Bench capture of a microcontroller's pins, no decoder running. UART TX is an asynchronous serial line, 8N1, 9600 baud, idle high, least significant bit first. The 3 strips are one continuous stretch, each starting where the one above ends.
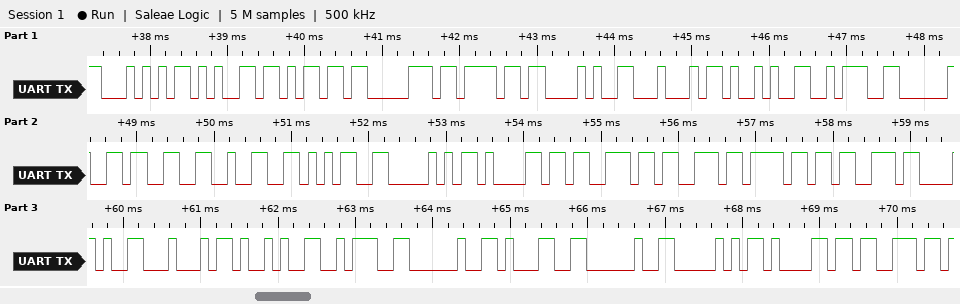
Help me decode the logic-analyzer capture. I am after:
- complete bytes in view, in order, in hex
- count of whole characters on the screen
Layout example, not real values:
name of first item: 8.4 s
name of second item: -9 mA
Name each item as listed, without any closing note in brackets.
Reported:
complete bytes in view, in order, in hex: 0x54 0x65 0x6D 0x70 0x6F 0x28 0x44 0x29 0x3A 0x20 0x33 0x32 0x35 0x50 0x61 0x73 0x73 0x6F 0x73 0x28 0x44 0x29 0x3A 0x20 0x31 0x20 0x50 0x61 0x73
count of whole characters on the screen: 29
